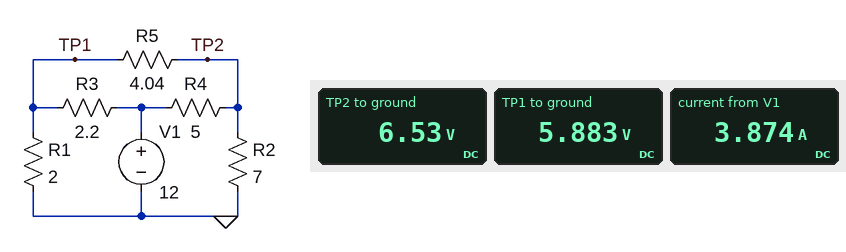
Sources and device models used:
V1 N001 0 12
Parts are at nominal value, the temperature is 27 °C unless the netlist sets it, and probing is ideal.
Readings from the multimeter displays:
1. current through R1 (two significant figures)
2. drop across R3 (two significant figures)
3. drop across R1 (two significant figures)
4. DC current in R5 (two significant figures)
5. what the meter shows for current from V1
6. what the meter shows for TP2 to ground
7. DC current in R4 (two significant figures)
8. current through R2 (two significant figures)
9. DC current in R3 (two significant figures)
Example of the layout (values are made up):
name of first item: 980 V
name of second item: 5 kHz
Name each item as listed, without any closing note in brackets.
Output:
current through R1: 2.9 A
drop across R3: 6.1 V
drop across R1: 5.9 V
DC current in R5: 160 mA
what the meter shows for current from V1: 3.874 A
what the meter shows for TP2 to ground: 6.53 V
DC current in R4: 1.1 A
current through R2: 930 mA
DC current in R3: 2.8 A
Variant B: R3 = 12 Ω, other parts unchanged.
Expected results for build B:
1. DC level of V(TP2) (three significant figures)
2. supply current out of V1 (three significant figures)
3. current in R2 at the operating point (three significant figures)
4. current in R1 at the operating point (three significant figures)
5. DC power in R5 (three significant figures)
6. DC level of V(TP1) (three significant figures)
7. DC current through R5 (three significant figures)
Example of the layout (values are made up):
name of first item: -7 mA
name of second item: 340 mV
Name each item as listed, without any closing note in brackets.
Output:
DC level of V(TP2): 5.22 V
supply current out of V1: 2.13 A
current in R2 at the operating point: 746 mA
current in R1 at the operating point: 1.38 A
DC power in R5: 1.50 W
DC level of V(TP1): 2.76 V
DC current through R5: 610 mA
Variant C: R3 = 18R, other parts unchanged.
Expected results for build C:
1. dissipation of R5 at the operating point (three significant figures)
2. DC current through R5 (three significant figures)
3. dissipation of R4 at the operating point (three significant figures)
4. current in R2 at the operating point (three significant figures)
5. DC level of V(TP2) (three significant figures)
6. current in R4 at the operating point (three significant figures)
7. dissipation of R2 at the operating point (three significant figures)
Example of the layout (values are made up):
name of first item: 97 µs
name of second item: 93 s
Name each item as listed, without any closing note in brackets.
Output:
dissipation of R5 at the operating point: 1.77 W
DC current through R5: 662 mA
dissipation of R4 at the operating point: 9.61 W
current in R2 at the operating point: 724 mA
DC level of V(TP2): 5.07 V
current in R4 at the operating point: 1.39 A
dissipation of R2 at the operating point: 3.67 W
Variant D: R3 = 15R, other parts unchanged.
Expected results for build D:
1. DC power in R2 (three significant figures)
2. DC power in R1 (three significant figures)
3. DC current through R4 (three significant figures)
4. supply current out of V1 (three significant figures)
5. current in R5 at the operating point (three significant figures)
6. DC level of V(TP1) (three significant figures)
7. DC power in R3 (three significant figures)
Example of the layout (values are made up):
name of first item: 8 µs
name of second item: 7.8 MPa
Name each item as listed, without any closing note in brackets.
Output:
DC power in R2: 3.76 W
DC power in R1: 3.23 W
DC current through R4: 1.37 A
supply current out of V1: 2.00 A
current in R5 at the operating point: 641 mA
DC level of V(TP1): 2.54 V
DC power in R3: 5.96 W
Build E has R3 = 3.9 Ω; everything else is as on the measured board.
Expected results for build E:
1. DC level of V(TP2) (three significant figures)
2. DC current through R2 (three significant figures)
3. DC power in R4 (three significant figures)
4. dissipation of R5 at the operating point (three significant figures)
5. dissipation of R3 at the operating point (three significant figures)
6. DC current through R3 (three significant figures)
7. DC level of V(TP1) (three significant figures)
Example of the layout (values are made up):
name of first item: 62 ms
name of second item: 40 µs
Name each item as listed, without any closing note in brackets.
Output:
DC level of V(TP2): 5.97 V
DC current through R2: 852 mA
DC power in R4: 7.28 W
dissipation of R5 at the operating point: 507 mW
dissipation of R3 at the operating point: 14.3 W
DC current through R3: 1.91 A
DC level of V(TP1): 4.54 V
